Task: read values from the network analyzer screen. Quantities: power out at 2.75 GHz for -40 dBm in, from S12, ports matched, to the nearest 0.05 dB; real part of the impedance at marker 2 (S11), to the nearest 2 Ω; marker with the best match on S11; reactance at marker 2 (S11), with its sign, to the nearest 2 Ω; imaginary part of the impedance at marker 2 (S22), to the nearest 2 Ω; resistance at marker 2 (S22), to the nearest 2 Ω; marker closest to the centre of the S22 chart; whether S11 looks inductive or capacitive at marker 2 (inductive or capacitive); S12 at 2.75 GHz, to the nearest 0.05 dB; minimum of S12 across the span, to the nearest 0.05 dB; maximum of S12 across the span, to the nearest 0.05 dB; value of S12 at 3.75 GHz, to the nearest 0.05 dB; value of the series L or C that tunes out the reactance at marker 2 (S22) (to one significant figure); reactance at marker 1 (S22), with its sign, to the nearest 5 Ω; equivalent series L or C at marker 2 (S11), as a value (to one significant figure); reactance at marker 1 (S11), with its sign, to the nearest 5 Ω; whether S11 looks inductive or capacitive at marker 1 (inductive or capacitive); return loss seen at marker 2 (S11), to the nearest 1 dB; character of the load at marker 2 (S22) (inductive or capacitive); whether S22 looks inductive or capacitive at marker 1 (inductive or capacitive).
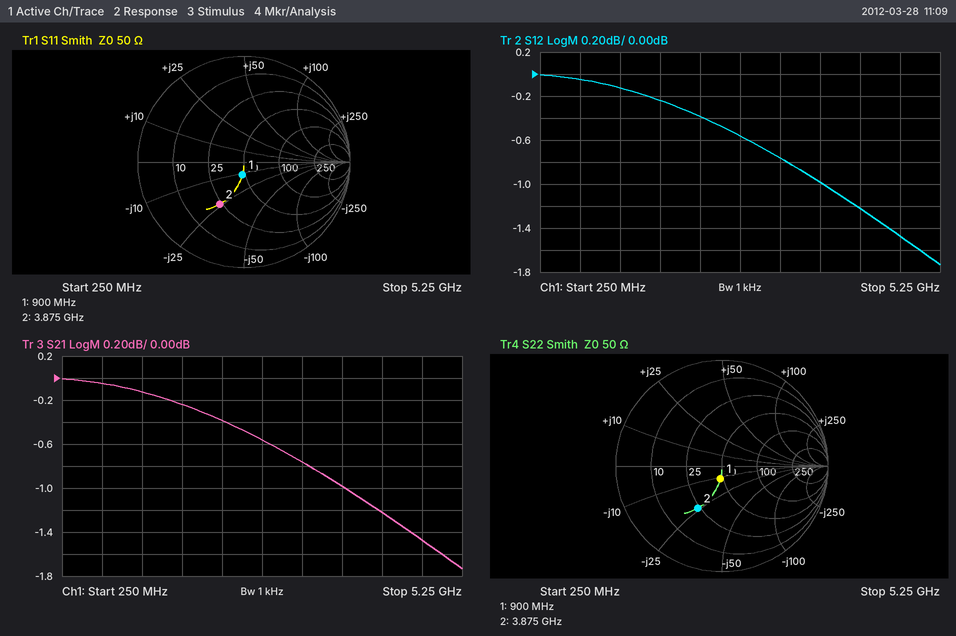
-40.55 dBm
24 Ω
marker 1
-24 Ω
-24 Ω
24 Ω
marker 1
capacitive
-0.55 dB
-1.75 dB
0.00 dB
-1.00 dB
1.0 nH
-10 Ω
2 pF
-10 Ω
capacitive
7 dB
capacitive
capacitive
